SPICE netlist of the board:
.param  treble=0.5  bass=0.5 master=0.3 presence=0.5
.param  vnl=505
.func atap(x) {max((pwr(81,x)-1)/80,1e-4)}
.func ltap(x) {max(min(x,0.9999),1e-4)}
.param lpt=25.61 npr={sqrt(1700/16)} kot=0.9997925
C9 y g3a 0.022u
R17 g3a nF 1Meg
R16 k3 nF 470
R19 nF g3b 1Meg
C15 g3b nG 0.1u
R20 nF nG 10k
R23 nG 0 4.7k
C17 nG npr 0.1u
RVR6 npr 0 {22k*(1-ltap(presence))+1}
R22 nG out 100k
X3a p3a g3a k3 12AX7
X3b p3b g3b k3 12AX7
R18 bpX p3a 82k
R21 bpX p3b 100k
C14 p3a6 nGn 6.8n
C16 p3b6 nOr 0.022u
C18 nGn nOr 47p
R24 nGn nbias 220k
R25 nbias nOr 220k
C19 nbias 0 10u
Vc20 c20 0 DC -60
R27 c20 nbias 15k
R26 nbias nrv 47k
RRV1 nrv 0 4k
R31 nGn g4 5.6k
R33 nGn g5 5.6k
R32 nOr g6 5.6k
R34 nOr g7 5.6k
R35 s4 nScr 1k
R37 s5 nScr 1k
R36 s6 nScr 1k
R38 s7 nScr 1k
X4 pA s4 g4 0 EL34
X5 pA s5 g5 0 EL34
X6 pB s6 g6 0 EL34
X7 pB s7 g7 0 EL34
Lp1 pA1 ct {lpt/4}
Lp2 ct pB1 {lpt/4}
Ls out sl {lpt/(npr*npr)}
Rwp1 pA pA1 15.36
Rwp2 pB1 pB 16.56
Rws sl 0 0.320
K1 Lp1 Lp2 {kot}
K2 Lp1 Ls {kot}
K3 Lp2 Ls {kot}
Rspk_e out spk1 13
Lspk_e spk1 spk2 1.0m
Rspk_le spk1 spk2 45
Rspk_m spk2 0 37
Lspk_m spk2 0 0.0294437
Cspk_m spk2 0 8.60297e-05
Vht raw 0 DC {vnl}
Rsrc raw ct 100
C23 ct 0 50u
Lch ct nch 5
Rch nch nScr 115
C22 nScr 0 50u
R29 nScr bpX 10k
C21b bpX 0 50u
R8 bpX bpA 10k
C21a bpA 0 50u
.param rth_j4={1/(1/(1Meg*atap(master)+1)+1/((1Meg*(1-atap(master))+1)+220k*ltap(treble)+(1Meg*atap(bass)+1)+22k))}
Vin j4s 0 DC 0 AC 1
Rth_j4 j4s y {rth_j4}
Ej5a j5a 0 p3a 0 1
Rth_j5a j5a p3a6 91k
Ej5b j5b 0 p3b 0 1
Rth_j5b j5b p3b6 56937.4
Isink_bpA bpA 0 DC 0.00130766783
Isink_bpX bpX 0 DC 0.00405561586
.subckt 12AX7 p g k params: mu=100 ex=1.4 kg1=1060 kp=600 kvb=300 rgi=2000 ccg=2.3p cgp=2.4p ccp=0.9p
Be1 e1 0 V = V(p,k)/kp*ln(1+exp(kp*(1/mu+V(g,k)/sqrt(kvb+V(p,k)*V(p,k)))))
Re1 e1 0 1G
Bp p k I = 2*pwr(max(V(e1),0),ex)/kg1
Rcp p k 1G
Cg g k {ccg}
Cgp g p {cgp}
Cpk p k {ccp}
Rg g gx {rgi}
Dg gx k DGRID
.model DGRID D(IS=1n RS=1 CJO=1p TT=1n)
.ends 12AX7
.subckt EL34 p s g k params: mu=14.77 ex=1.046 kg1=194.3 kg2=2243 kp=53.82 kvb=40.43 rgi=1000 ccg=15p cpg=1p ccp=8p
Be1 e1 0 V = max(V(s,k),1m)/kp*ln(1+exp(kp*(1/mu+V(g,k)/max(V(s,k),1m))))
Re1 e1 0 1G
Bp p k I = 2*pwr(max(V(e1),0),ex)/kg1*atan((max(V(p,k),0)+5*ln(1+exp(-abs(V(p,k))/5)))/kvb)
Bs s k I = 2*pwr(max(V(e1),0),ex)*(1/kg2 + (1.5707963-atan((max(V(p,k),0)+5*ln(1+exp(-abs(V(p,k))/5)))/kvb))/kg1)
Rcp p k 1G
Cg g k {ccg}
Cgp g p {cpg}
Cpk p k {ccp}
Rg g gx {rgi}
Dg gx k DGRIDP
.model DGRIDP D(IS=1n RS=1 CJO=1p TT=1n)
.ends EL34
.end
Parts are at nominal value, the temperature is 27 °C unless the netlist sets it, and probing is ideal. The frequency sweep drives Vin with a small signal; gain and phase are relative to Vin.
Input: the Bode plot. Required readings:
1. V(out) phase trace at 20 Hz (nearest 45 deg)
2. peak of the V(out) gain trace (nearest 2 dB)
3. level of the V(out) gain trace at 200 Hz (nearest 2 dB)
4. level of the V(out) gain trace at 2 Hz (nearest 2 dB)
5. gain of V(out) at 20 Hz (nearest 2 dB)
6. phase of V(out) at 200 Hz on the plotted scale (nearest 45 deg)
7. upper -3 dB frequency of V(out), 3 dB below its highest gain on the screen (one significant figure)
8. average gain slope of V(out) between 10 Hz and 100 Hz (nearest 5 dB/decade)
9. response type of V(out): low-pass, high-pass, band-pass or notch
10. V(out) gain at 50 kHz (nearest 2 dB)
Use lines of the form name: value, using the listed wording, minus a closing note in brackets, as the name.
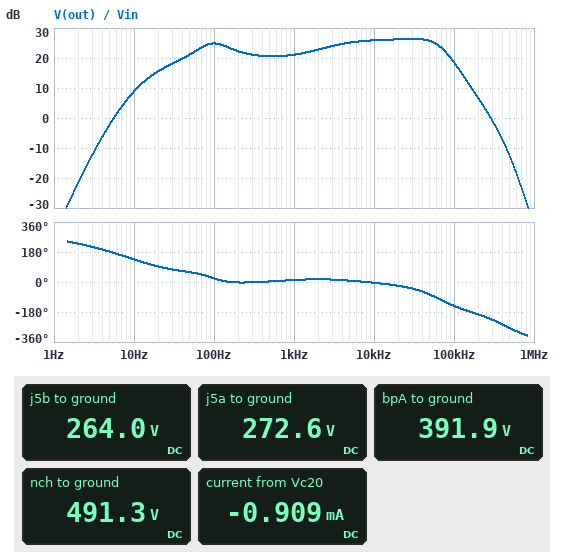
V(out) phase trace at 20 Hz: 90 deg
peak of the V(out) gain trace: 26 dB
level of the V(out) gain trace at 200 Hz: 22 dB
level of the V(out) gain trace at 2 Hz: -22 dB
gain of V(out) at 20 Hz: 16 dB
phase of V(out) at 200 Hz on the plotted scale: 0 deg
upper -3 dB frequency of V(out), 3 dB below its highest gain on the screen: 70 kHz
average gain slope of V(out) between 10 Hz and 100 Hz: 15 dB/decade
response type of V(out): low-pass, high-pass, band-pass or notch: band-pass
V(out) gain at 50 kHz: 26 dB
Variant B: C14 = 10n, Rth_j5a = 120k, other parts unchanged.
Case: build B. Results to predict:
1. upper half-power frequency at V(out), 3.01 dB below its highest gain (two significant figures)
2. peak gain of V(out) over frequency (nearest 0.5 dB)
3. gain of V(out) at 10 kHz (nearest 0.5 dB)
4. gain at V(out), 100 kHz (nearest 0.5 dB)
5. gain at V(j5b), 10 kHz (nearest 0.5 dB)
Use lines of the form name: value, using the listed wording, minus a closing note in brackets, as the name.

upper half-power frequency at V(out), 3.01 dB below its highest gain: 64 kHz
peak gain of V(out) over frequency: 26.0 dB
gain of V(out) at 10 kHz: 25.5 dB
gain at V(out), 100 kHz: 17.5 dB
gain at V(j5b), 10 kHz: 21.0 dB
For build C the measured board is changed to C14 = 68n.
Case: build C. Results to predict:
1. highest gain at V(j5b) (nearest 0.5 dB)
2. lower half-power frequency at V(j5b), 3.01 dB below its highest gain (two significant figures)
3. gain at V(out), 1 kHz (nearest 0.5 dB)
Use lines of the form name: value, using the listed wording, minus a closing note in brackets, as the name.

highest gain at V(j5b): 28.5 dB
lower half-power frequency at V(j5b), 3.01 dB below its highest gain: 3.5 Hz
gain at V(out), 1 kHz: 21.0 dB
